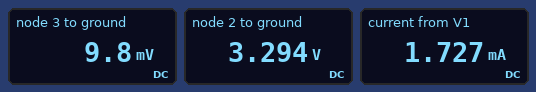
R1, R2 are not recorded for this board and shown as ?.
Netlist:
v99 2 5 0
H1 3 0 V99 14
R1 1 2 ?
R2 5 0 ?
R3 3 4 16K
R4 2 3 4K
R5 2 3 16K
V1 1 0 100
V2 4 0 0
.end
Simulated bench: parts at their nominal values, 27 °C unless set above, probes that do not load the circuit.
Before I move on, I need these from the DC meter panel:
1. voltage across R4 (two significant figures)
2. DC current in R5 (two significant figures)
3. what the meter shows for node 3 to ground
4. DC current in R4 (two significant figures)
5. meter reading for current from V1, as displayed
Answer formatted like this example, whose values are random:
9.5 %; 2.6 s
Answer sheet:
3.3 V; 210 µA; 9.8 mV; 820 µA; 1.727 mA
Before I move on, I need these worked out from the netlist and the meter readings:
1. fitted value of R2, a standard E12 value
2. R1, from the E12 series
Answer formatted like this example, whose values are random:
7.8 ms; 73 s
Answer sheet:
4.7 kΩ; 56 kΩ
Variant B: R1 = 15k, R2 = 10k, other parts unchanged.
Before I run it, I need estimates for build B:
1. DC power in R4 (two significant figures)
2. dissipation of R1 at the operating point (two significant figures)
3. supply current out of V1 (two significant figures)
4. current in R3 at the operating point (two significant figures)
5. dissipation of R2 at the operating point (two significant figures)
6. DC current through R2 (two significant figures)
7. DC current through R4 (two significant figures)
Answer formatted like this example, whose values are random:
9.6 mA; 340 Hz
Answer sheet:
48 mW; 490 mW; 5.7 mA; 1.2 µA; 19 mW; 1.4 mA; 3.5 mA
